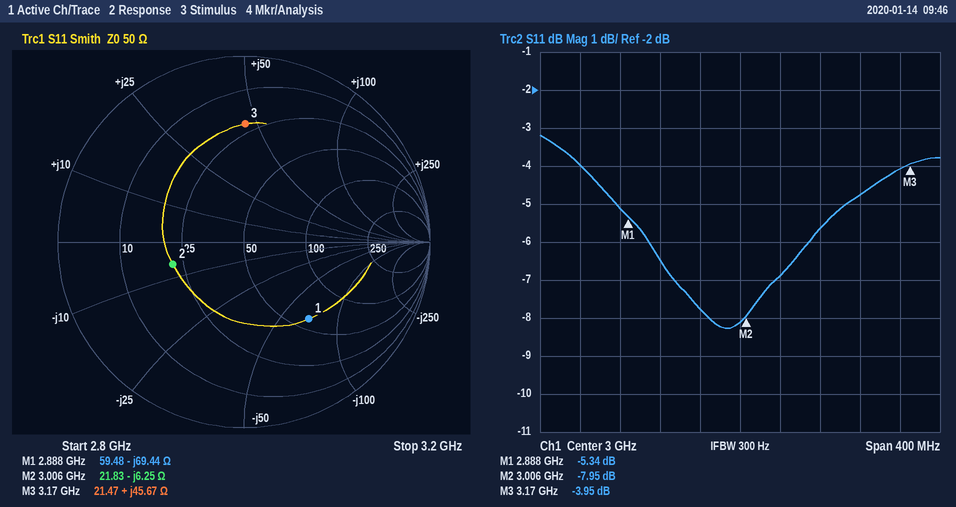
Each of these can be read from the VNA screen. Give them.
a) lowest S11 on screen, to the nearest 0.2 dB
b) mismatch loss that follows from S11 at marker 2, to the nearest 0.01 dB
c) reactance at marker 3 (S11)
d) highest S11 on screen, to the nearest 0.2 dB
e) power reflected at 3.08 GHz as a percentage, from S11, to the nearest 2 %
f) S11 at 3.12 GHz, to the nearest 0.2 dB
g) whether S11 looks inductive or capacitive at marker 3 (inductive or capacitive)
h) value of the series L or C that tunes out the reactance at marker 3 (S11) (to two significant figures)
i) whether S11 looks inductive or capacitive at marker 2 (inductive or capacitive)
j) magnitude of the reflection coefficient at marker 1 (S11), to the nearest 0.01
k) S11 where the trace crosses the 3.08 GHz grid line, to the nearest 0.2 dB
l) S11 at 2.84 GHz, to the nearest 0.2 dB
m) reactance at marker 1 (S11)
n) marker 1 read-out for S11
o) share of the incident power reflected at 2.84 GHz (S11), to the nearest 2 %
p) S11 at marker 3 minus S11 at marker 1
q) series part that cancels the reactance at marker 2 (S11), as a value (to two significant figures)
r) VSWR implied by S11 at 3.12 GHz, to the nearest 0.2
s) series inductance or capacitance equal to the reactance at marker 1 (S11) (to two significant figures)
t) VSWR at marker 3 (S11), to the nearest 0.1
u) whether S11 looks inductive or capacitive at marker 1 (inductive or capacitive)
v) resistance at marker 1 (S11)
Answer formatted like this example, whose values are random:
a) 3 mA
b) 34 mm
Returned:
a) -8.2 dB
b) 0.76 dB
c) +45.67 Ω
d) -3.2 dB
e) 28 %
f) -4.8 dB
g) inductive
h) 1.1 pF
i) capacitive
j) 0.54
k) -5.6 dB
l) -4.0 dB
m) -69.44 Ω
n) -5.34 dB
o) 40 %
p) 1.39 dB
q) 330 pH
r) 3.8
s) 790 fF
t) 4.5
u) capacitive
v) 59.48 Ω
